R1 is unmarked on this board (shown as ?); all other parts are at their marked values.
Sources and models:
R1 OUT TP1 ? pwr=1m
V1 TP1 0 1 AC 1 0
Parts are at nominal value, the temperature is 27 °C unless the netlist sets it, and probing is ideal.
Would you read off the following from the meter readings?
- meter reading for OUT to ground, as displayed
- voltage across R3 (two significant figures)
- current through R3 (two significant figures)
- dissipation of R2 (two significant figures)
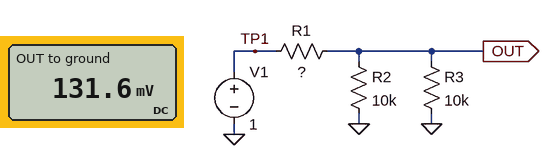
131.6 mV
130 mV
13 µA
1.7 µW
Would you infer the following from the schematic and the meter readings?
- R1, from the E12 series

33 kΩ
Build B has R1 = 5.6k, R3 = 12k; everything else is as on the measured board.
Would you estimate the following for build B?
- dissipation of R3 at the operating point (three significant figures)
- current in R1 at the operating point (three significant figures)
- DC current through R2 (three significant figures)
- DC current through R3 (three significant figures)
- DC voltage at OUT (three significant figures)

20.3 µW
90.5 µA
49.3 µA
41.1 µA
493 mV
